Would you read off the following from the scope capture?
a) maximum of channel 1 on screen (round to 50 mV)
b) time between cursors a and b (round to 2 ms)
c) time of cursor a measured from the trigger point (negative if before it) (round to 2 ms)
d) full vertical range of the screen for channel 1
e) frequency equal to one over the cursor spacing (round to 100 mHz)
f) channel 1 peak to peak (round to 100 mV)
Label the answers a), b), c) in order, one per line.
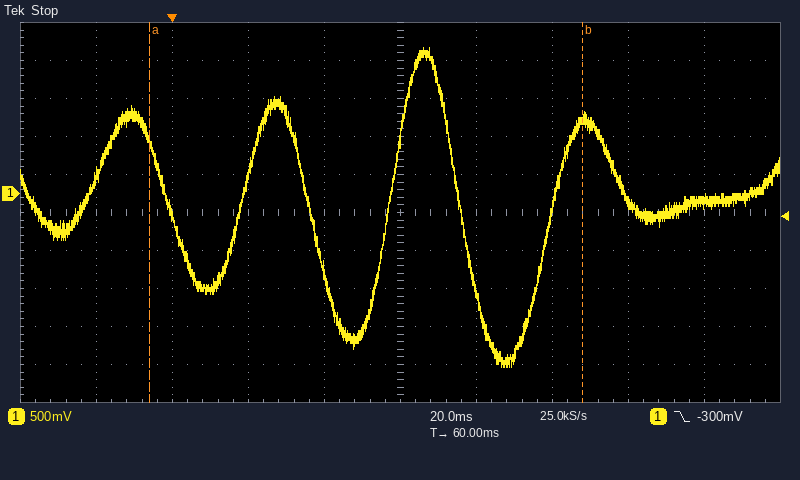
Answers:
a) 1.90 V
b) 114 ms
c) -6 ms
d) 5 V
e) 8.8 Hz
f) 4.20 V
